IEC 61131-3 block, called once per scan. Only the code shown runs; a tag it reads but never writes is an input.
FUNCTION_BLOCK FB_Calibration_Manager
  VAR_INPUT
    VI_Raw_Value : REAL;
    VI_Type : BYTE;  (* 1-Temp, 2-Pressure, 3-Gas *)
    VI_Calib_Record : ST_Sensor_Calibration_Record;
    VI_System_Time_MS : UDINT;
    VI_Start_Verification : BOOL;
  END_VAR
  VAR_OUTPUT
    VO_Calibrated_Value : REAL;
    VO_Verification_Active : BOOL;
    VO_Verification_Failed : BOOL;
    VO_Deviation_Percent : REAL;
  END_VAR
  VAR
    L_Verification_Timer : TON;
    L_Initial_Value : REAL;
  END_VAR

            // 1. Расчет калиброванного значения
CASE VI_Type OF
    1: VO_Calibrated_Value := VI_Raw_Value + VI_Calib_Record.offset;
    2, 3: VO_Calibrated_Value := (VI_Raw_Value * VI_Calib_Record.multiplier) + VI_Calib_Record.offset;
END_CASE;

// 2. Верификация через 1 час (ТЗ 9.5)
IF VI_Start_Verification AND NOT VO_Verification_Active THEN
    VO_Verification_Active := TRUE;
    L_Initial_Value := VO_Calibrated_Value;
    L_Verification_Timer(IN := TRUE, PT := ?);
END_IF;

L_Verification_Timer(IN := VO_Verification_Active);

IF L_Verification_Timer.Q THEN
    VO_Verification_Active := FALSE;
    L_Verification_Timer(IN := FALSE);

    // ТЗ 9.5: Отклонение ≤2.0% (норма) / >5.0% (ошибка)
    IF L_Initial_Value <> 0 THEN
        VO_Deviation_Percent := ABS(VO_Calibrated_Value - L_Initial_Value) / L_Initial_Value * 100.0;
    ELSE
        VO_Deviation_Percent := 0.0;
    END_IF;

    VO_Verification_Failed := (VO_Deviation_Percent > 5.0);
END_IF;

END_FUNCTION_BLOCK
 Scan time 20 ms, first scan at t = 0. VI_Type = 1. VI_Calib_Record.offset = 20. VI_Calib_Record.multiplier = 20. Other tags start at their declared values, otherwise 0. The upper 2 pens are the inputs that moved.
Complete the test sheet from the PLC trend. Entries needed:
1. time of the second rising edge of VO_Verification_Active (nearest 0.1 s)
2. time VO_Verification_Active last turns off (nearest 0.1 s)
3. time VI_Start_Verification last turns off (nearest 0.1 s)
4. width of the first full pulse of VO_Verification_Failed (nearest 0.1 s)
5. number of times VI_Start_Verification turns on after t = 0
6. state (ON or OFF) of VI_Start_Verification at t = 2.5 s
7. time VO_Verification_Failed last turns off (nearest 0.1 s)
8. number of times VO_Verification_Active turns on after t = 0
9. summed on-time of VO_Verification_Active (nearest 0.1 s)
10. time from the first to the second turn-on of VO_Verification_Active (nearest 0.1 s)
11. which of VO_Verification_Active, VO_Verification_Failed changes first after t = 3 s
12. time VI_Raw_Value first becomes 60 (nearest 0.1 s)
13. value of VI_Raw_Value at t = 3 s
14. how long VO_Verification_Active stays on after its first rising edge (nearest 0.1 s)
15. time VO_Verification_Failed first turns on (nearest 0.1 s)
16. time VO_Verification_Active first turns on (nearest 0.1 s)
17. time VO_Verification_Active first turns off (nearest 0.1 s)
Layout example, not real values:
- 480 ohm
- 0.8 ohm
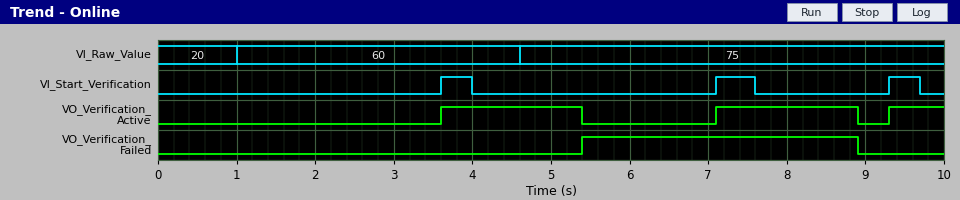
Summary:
- 7.1 s
- 8.9 s
- 9.7 s
- 3.5 s
- 3
- OFF
- 8.9 s
- 3
- 4.3 s
- 3.5 s
- VO_Verification_Active
- 1.0 s
- 60
- 1.8 s
- 5.4 s
- 3.6 s
- 5.4 s
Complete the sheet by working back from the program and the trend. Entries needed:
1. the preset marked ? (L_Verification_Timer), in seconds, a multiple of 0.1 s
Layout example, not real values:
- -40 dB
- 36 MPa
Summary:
- 1.8 s
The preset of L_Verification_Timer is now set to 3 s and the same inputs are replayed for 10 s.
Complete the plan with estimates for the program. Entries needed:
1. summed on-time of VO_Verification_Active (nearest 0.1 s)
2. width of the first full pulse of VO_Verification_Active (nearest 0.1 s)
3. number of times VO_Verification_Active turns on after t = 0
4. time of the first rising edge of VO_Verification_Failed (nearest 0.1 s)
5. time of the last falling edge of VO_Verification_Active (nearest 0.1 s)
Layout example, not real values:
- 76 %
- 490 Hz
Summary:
- 5.9 s
- 3.0 s
- 2
- 6.6 s
- 6.6 s
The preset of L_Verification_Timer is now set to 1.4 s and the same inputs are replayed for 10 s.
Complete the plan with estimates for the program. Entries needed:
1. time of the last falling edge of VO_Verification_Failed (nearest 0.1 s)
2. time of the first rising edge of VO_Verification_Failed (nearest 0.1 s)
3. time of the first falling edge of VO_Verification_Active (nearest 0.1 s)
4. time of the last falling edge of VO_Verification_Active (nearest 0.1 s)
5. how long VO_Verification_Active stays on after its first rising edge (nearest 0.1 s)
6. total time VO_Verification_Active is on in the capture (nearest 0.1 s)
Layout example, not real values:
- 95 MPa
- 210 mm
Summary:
- 8.5 s
- 5.0 s
- 5.0 s
- 8.5 s
- 1.4 s
- 3.5 s
